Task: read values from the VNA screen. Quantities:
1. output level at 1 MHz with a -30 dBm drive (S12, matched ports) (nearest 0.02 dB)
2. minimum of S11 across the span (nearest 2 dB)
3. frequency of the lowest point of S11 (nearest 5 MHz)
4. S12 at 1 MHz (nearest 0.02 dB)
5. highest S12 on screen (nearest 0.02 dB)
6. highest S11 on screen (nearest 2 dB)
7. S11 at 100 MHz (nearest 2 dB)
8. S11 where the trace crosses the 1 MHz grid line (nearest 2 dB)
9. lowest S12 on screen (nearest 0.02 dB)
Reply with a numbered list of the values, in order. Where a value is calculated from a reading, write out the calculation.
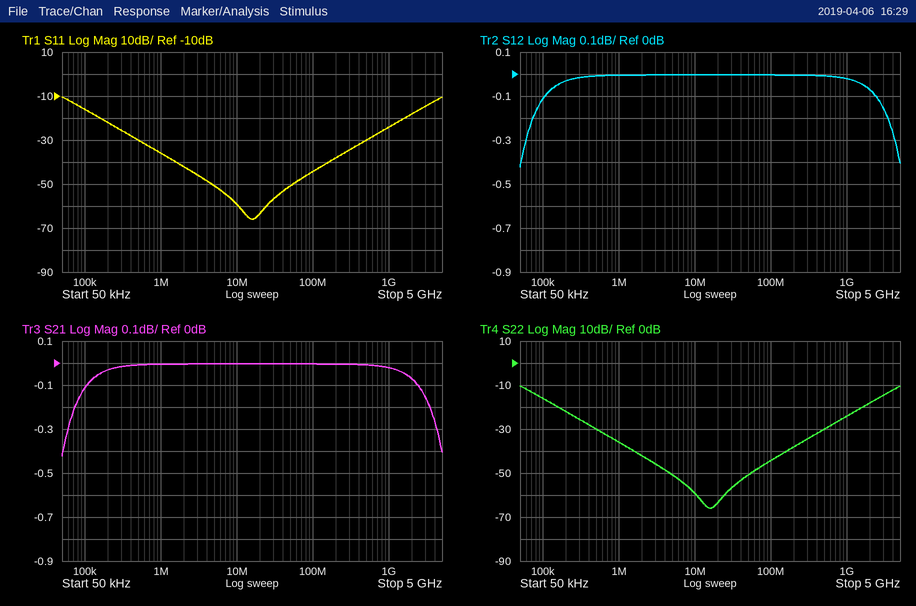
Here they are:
1. -30 dBm + (0.00 dB) = -30.00 dBm
2. -66 dB
3. 15 MHz
4. 0.00 dB
5. 0.00 dB
6. -10 dB
7. -44 dB
8. -36 dB
9. -0.42 dB
